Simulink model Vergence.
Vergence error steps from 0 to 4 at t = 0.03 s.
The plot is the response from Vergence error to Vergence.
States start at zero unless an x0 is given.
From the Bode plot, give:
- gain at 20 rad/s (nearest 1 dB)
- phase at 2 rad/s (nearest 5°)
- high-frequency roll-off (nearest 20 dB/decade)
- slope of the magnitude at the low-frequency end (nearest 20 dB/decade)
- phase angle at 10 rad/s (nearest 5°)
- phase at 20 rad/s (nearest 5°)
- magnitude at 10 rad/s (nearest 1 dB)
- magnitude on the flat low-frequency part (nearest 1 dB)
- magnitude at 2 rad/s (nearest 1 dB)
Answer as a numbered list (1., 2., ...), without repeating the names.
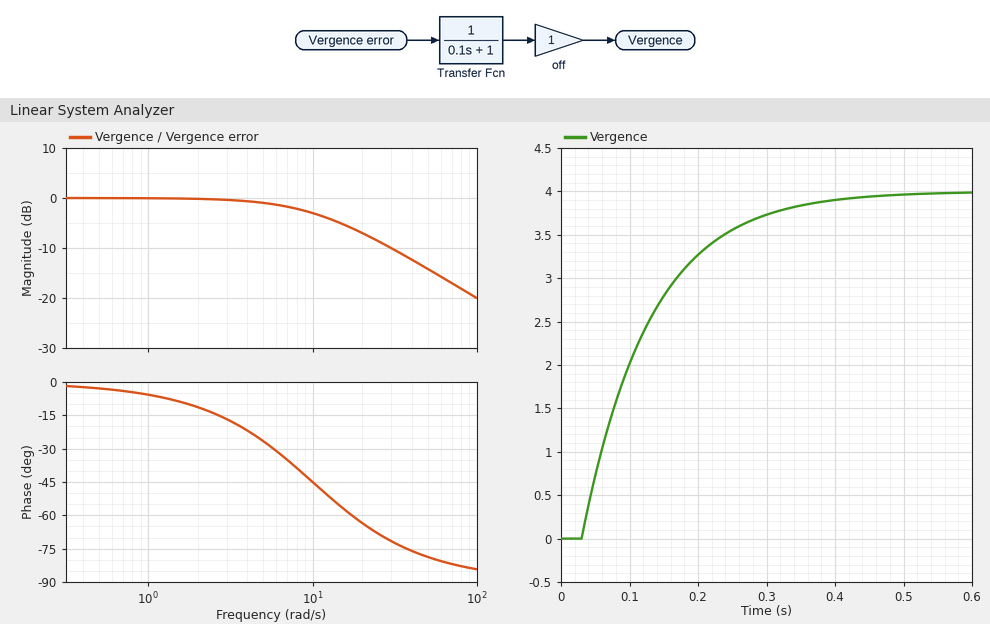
1. -7 dB
2. -10°
3. -20 dB/decade
4. 0 dB/decade
5. -45°
6. -65°
7. -3 dB
8. 0 dB
9. 0 dB
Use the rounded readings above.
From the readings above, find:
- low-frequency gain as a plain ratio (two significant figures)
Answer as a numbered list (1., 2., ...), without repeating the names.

1. 1.0
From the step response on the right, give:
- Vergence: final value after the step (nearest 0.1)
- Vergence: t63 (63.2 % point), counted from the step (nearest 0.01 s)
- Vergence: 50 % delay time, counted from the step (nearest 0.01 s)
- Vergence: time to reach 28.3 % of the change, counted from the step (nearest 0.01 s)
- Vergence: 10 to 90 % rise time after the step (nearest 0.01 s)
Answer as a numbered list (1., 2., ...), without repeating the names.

1. 4.0
2. 0.10 s
3. 0.07 s
4. 0.03 s
5. 0.22 s
